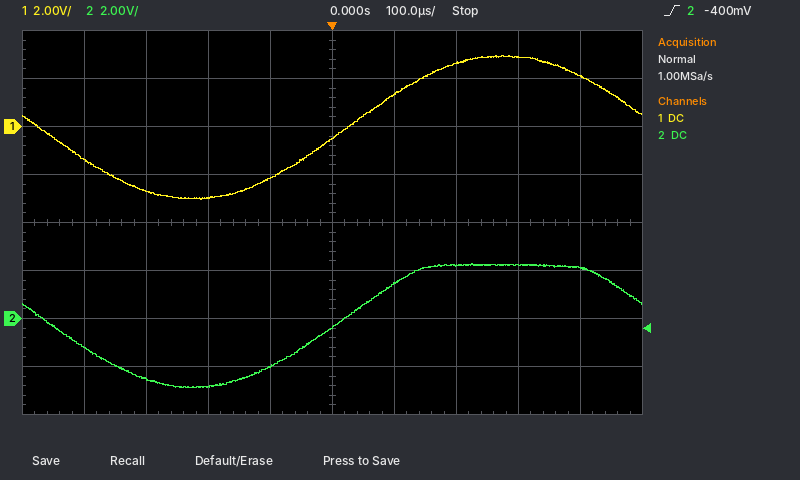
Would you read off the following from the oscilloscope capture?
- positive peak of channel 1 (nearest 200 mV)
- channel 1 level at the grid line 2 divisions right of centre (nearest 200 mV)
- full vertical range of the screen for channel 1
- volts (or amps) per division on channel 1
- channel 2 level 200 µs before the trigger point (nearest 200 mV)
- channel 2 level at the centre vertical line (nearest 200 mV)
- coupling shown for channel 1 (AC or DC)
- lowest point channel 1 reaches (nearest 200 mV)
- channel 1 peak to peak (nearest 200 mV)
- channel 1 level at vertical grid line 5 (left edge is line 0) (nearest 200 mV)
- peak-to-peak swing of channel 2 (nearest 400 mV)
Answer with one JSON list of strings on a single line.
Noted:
["3.0 V", "2.6 V", "16 V", "2 V", "-2.8 V", "-400 mV", "DC", "-3.0 V", "6.0 V", "-600 mV", "5.2 V"]
